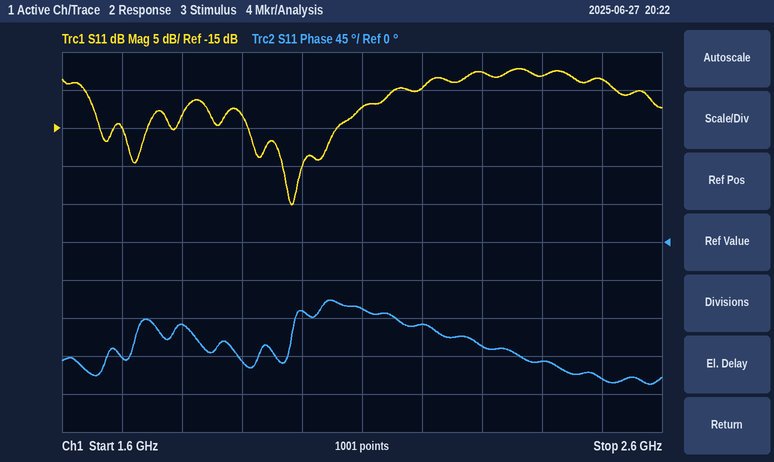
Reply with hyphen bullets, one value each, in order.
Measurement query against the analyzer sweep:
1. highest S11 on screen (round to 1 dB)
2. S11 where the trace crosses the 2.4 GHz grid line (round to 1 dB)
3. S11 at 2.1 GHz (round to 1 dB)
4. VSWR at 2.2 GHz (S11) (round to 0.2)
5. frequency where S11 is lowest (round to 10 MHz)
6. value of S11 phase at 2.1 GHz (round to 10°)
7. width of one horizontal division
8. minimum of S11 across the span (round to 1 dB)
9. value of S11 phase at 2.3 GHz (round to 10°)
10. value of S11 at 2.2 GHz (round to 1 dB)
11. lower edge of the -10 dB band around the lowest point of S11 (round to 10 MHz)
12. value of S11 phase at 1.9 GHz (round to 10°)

- -7 dB
- -8 dB
- -12 dB
- 2.0
- 1.98 GHz
- -80°
- 100 MHz
- -25 dB
- -120°
- -10 dB
- 1.64 GHz
- -140°
